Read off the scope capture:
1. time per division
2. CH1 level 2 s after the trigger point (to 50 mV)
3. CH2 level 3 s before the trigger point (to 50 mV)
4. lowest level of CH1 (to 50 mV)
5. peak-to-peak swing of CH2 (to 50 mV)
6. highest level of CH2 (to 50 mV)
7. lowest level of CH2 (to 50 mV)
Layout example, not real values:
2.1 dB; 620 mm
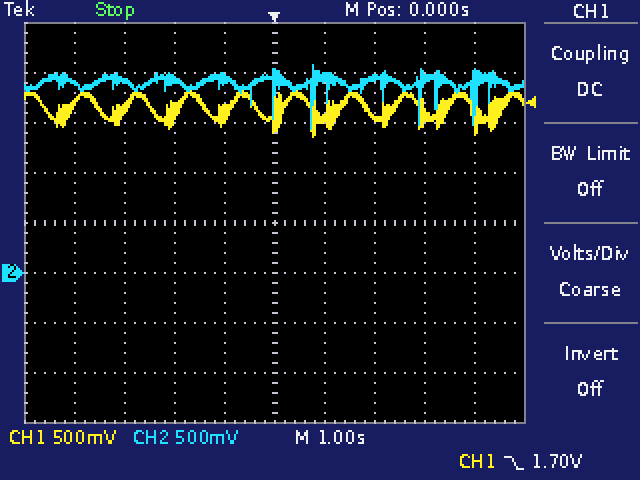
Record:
1 s; 1.55 V; 1.95 V; 1.35 V; 650 mV; 2.10 V; 1.45 V
